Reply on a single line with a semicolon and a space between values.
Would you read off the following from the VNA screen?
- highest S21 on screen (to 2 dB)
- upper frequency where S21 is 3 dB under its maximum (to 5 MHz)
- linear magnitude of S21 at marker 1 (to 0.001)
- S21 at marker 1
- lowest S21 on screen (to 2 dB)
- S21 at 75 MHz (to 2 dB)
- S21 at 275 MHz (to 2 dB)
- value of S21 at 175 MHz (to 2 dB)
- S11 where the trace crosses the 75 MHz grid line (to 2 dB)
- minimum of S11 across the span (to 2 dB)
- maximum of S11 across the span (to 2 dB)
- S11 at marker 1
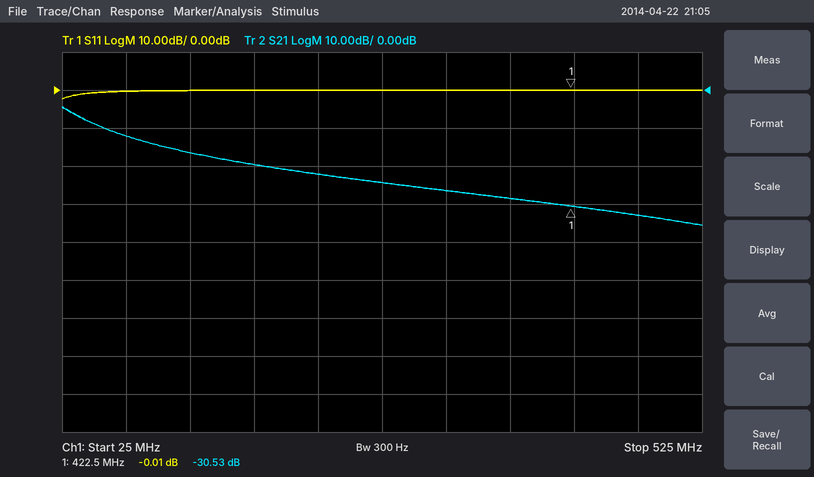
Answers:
-4 dB; 40 MHz; 0.030; -30.53 dB; -36 dB; -12 dB; -24 dB; -20 dB; 0 dB; -2 dB; 0 dB; -0.01 dB
